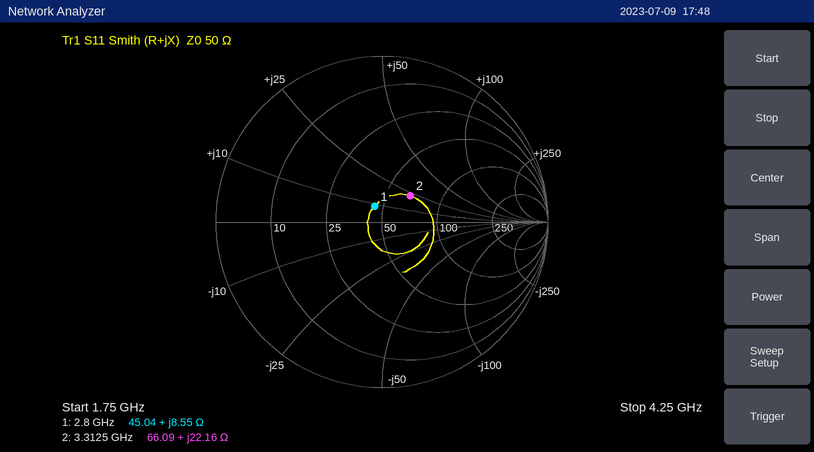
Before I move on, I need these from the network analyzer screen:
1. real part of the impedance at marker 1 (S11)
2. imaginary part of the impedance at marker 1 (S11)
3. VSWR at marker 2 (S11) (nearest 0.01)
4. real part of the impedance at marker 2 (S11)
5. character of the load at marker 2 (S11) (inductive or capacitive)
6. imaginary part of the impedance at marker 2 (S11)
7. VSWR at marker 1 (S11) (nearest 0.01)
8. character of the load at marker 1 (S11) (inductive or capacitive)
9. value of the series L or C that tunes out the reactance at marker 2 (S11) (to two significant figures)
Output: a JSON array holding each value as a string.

["45.04 Ω", "+8.55 Ω", "1.60", "66.09 Ω", "inductive", "+22.16 Ω", "1.23", "inductive", "2.2 pF"]
